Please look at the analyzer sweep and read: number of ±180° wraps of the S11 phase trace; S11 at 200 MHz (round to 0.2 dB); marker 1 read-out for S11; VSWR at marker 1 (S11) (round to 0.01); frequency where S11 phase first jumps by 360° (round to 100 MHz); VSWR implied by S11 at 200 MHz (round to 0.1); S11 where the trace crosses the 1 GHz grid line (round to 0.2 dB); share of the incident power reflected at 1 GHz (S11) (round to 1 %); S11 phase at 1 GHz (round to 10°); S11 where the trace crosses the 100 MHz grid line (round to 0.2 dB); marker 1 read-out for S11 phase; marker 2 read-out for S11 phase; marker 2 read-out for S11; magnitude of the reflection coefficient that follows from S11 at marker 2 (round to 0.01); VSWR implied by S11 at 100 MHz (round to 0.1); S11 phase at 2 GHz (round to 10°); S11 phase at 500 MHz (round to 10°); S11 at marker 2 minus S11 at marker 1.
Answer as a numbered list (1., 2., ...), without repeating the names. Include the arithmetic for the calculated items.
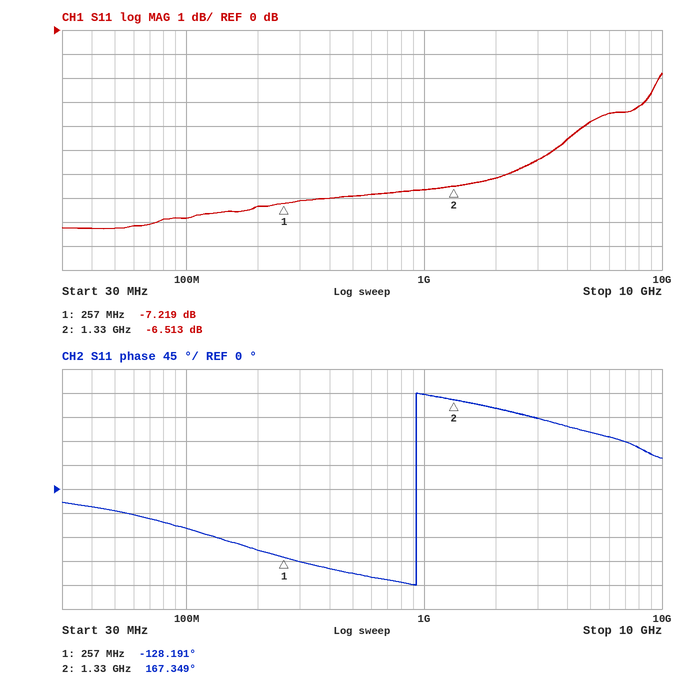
1. 1
2. -7.4 dB
3. -7.219 dB
4. (1 + 0.4356)/(1 − 0.4356) ≈ 2.54
5. 900 MHz
6. |Γ| = 10^(-7.4/20) = 0.4266; VSWR = (1 + 0.4266)/(1 − 0.4266) ≈ 2.5
7. -6.6 dB
8. 10^(-6.6/10) ≈ 22 %
9. 180°
10. -7.8 dB
11. -128.191°
12. 167.349°
13. -6.513 dB
14. 10^(-6.513/20) ≈ 0.47
15. |Γ| = 10^(-7.8/20) = 0.4074; VSWR = (1 + 0.4074)/(1 − 0.4074) ≈ 2.4
16. 150°
17. -160°
18. -6.513 − (-7.219) = 0.706 dB
